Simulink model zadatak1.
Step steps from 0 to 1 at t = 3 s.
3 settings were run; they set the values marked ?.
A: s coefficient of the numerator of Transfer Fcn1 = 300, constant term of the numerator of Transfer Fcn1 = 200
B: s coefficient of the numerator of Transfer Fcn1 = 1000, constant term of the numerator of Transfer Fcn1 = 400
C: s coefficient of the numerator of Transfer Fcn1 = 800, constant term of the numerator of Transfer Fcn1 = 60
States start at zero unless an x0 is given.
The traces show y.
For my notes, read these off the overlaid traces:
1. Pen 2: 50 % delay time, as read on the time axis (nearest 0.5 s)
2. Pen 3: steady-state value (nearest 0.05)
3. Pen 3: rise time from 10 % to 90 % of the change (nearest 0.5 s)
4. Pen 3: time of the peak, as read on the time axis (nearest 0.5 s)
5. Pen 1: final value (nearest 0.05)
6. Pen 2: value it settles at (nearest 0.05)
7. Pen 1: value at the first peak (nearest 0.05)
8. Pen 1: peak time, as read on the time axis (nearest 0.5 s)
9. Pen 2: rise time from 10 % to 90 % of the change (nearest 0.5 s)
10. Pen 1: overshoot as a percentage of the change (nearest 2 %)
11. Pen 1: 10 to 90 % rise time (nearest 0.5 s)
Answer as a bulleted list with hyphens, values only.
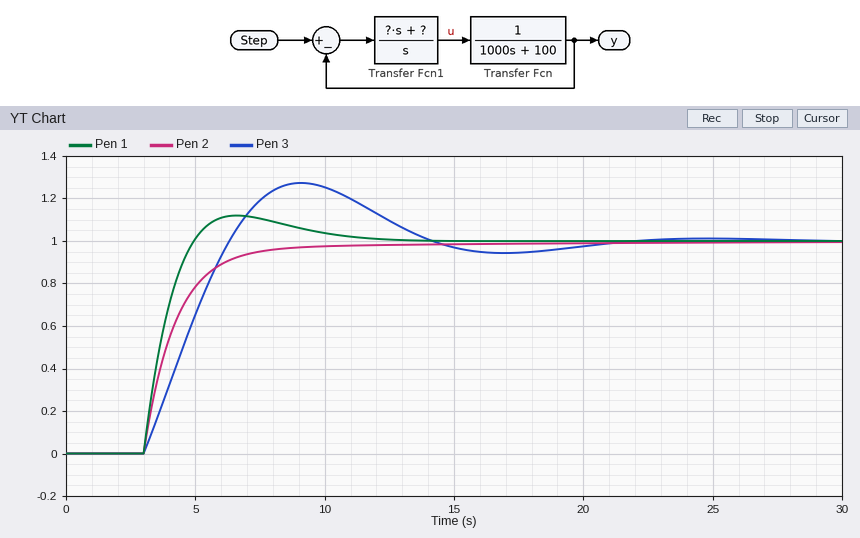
- 4.0 s
- 1.00
- 2.5 s
- 9.0 s
- 1.00
- 1.00
- 1.10
- 6.5 s
- 3.0 s
- 12 %
- 1.5 s
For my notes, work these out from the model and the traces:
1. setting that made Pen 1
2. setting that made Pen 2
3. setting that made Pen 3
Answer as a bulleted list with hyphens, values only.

- B
- C
- A
